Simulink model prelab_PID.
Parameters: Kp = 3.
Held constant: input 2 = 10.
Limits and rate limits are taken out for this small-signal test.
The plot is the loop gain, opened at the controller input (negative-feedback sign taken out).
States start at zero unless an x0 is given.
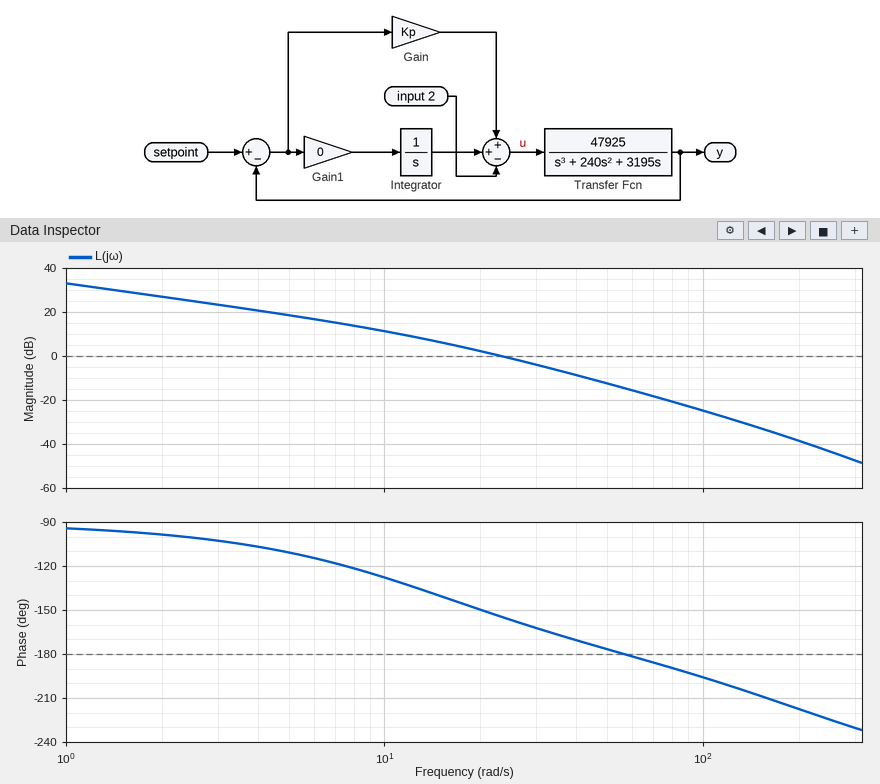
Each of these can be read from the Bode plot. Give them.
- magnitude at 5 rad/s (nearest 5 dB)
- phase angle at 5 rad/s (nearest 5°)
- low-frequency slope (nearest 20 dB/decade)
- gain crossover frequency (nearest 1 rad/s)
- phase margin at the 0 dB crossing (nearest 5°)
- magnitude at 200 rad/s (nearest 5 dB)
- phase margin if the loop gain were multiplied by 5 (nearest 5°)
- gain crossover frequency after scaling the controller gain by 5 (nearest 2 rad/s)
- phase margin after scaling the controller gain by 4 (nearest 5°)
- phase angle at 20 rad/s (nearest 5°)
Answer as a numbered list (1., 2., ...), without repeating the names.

1. 20 dB
2. -110°
3. -20 dB/decade
4. 23 rad/s
5. 25°
6. -40 dB
7. 0°
8. 54 rad/s
9. 5°
10. -150°
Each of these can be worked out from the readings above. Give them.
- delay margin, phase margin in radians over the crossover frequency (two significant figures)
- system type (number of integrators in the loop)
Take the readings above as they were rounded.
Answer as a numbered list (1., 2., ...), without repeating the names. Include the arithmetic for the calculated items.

1. 25 × π / 180 / 23 = 0.019 s
2. 1
